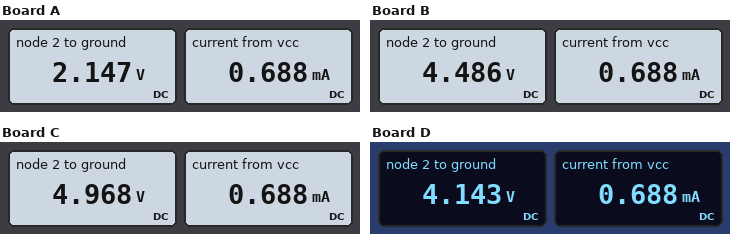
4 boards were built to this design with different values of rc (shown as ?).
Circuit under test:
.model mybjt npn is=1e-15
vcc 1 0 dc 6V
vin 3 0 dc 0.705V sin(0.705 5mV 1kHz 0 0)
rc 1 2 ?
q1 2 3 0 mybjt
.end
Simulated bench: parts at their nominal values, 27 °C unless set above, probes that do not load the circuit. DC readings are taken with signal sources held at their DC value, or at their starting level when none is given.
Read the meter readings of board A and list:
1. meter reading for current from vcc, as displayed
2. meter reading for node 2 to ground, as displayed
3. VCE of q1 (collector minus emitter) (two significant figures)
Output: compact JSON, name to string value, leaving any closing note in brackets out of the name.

{"meter reading for current from vcc, as displayed": "0.688 mA", "meter reading for node 2 to ground, as displayed": "2.147 V", "VCE of q1 (collector minus emitter)": "2.1 V"}
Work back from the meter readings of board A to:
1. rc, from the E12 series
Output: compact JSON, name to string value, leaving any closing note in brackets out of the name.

{"rc, from the E12 series": "5.6 kΩ"}
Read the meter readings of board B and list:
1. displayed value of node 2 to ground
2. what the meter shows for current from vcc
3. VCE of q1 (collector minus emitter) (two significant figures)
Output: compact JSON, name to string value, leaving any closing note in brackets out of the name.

{"displayed value of node 2 to ground": "4.486 V", "what the meter shows for current from vcc": "0.688 mA", "VCE of q1 (collector minus emitter)": "4.5 V"}
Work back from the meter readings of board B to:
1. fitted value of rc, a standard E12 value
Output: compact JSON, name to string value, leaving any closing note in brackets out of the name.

{"fitted value of rc, a standard E12 value": "2.2 kΩ"}
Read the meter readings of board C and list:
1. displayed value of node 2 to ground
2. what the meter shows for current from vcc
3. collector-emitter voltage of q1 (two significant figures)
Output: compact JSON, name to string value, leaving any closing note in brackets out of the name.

{"displayed value of node 2 to ground": "4.968 V", "what the meter shows for current from vcc": "0.688 mA", "collector-emitter voltage of q1": "5.0 V"}
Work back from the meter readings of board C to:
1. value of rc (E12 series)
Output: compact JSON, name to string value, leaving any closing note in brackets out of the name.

{"value of rc": "1.5 kΩ"}
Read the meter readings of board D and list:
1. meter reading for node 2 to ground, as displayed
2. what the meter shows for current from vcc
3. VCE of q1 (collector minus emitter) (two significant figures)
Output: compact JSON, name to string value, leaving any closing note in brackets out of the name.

{"meter reading for node 2 to ground, as displayed": "4.143 V", "what the meter shows for current from vcc": "0.688 mA", "VCE of q1 (collector minus emitter)": "4.1 V"}
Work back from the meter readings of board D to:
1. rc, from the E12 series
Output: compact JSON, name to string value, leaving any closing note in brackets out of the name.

{"rc, from the E12 series": "2.7 kΩ"}
